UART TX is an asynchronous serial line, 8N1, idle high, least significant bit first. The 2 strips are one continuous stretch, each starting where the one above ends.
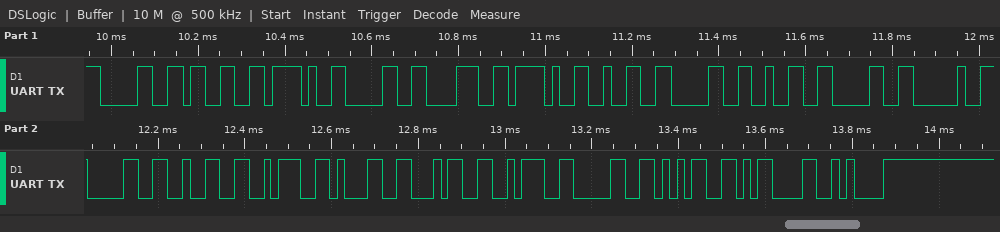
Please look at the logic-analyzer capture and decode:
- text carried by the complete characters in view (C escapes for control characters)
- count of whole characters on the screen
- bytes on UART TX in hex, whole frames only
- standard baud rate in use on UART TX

"03/08/2020 02:14:05\r\n"
21
30 33 2F 30 38 2F 32 30 32 30 20 30 32 3A 31 34 3A 30 35 0D 0A
57600 baud
